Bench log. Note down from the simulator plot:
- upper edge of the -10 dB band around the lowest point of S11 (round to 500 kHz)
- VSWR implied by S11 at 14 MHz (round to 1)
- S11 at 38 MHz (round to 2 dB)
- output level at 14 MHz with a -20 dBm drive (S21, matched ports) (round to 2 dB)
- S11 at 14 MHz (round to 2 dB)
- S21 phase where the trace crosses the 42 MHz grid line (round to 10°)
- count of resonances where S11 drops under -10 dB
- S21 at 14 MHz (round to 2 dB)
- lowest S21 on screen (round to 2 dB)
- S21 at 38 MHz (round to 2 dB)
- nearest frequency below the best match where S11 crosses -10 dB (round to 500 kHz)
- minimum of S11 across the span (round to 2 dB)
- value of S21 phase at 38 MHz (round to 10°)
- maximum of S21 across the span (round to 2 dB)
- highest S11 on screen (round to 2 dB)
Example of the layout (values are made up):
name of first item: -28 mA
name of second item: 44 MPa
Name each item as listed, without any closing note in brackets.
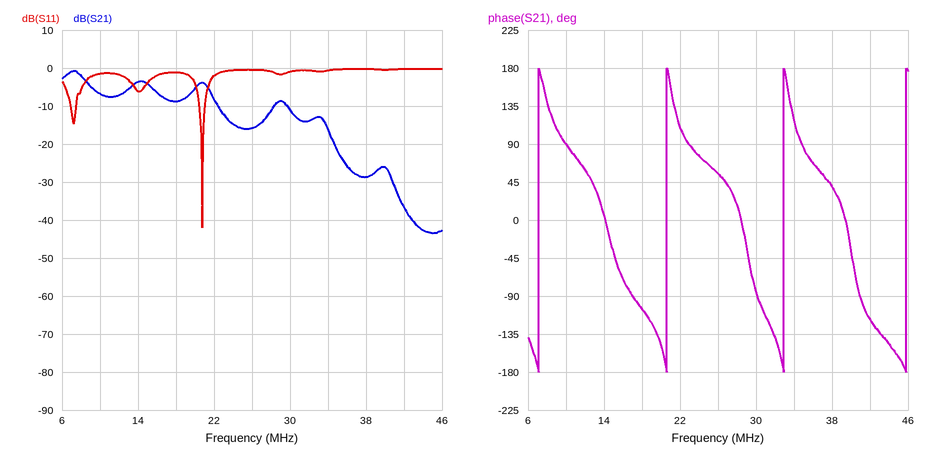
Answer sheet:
upper edge of the -10 dB band around the lowest point of S11: 21.0 MHz
VSWR implied by S11 at 14 MHz: 3
S11 at 38 MHz: 0 dB
output level at 14 MHz with a -20 dBm drive (S21, matched ports): -24 dBm
S11 at 14 MHz: -6 dB
S21 phase where the trace crosses the 42 MHz grid line: -120°
count of resonances where S11 drops under -10 dB: 2
S21 at 14 MHz: -4 dB
lowest S21 on screen: -44 dB
S21 at 38 MHz: -28 dB
nearest frequency below the best match where S11 crosses -10 dB: 20.5 MHz
minimum of S11 across the span: -42 dB
value of S21 phase at 38 MHz: 40°
maximum of S21 across the span: 0 dB
highest S11 on screen: 0 dB
